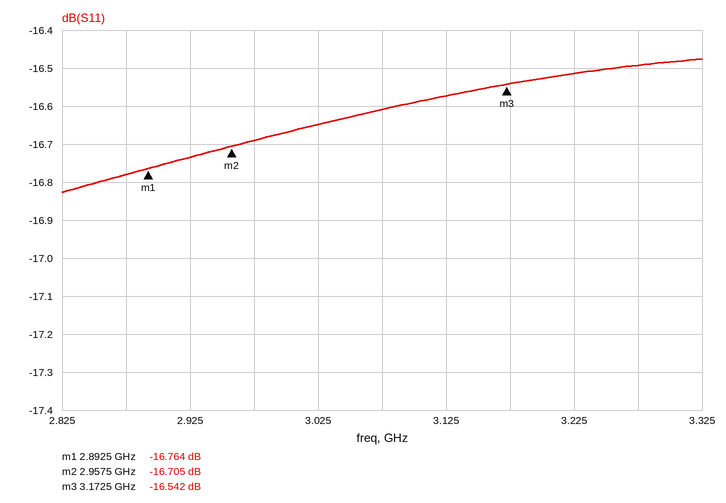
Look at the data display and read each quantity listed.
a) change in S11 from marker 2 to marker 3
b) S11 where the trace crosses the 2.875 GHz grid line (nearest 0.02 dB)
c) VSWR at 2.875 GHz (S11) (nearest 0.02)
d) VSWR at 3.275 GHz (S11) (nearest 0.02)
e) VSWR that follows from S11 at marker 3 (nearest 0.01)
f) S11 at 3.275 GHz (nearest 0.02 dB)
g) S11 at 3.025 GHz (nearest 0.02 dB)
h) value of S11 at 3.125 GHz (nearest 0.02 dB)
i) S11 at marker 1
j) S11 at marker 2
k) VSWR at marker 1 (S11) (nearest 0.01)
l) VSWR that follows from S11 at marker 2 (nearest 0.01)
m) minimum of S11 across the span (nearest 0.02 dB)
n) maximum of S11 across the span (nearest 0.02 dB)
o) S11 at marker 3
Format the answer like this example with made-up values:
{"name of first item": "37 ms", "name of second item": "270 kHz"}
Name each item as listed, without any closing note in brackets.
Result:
{"change in S11 from marker 2 to marker 3": "0.163 dB", "S11 where the trace crosses the 2.875 GHz grid line": "-16.78 dB", "VSWR at 2.875 GHz (S11)": "1.34", "VSWR at 3.275 GHz (S11)": "1.36", "VSWR that follows from S11 at marker 3": "1.35", "S11 at 3.275 GHz": "-16.50 dB", "S11 at 3.025 GHz": "-16.64 dB", "value of S11 at 3.125 GHz": "-16.58 dB", "S11 at marker 1": "-16.764 dB", "S11 at marker 2": "-16.705 dB", "VSWR at marker 1 (S11)": "1.34", "VSWR that follows from S11 at marker 2": "1.34", "minimum of S11 across the span": "-16.82 dB", "maximum of S11 across the span": "-16.48 dB", "S11 at marker 3": "-16.542 dB"}
